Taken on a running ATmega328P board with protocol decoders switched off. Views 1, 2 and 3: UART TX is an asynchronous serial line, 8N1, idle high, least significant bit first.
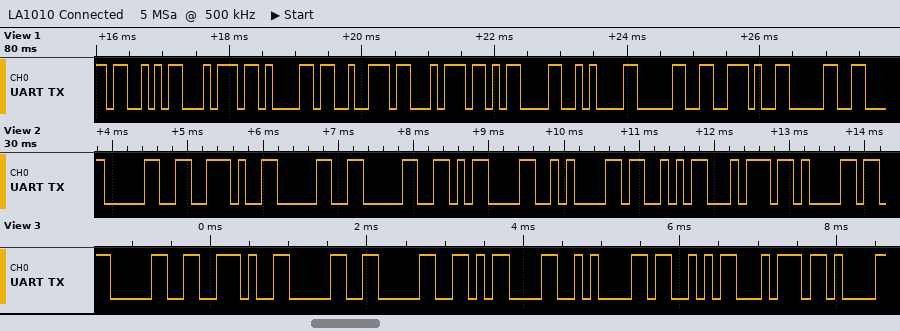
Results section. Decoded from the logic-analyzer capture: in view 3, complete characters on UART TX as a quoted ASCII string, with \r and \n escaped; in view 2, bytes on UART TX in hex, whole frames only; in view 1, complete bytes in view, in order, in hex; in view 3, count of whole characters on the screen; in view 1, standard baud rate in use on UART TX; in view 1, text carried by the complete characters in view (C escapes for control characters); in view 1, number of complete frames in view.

"0.00\r\nSt"
0x30 0x2E 0x30 0x30 0x0D 0x0A 0x53 0x74 0x61
53 74 61 72 74 0D 0A 30 2E 30
8
9600 baud
"Start\r\n0.0"
10
